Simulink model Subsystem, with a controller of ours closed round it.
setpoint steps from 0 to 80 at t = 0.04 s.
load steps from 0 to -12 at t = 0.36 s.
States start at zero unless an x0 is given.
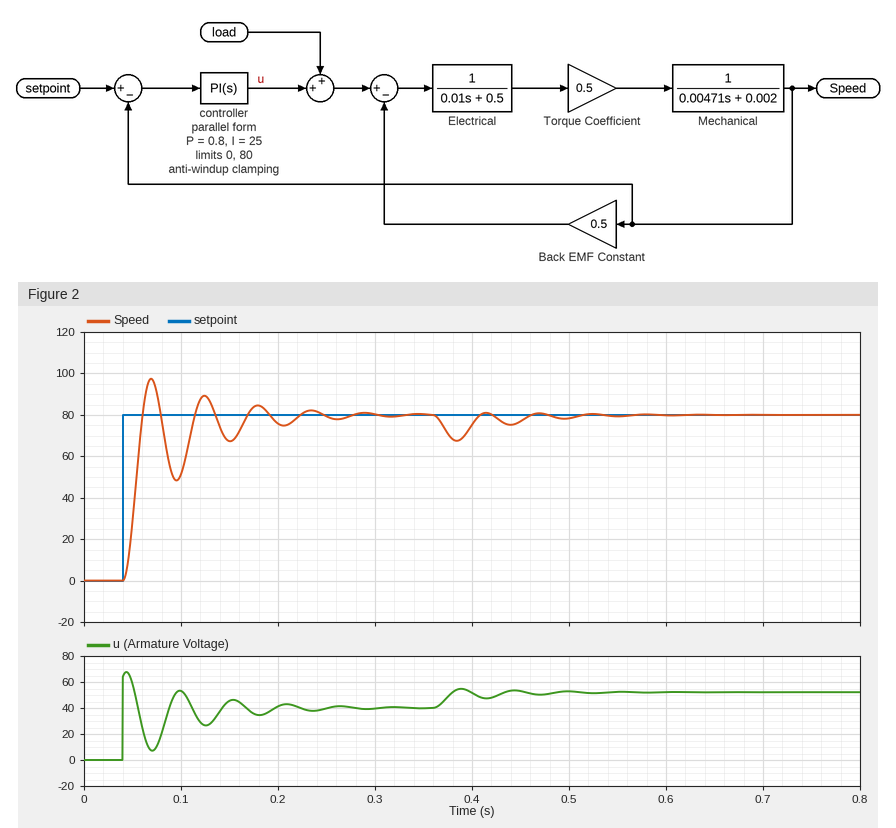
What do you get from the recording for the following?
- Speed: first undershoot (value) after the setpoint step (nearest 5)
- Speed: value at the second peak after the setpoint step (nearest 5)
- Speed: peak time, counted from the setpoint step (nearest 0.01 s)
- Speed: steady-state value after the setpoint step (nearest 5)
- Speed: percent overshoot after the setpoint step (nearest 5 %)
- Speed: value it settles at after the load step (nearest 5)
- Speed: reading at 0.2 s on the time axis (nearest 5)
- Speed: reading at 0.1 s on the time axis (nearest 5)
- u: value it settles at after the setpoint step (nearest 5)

50
90
0.03 s
80
20 %
80
75
50
40
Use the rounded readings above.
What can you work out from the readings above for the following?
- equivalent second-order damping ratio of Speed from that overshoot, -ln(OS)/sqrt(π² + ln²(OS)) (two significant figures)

0.46
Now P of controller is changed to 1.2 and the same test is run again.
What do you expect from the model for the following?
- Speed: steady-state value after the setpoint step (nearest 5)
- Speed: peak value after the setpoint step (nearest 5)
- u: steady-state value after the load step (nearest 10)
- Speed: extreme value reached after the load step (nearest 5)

80
95
50
70
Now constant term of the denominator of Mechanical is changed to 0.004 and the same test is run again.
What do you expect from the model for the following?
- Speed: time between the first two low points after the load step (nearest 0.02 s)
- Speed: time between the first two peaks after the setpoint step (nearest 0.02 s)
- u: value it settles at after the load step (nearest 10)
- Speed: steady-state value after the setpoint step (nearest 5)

0.06 s
0.06 s
50
80
